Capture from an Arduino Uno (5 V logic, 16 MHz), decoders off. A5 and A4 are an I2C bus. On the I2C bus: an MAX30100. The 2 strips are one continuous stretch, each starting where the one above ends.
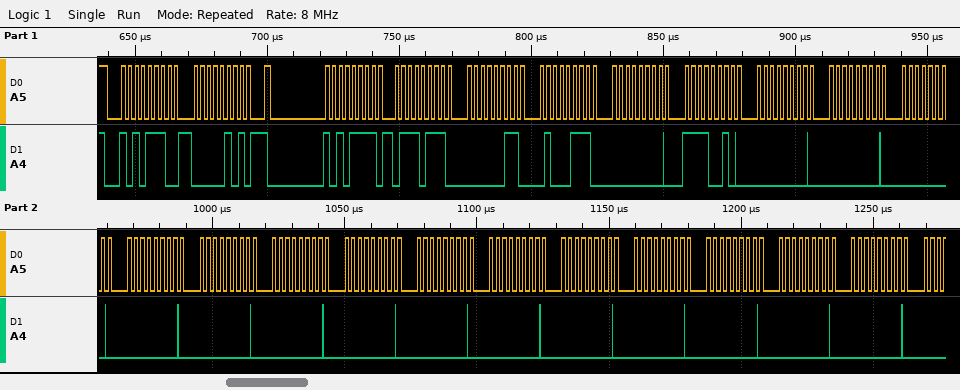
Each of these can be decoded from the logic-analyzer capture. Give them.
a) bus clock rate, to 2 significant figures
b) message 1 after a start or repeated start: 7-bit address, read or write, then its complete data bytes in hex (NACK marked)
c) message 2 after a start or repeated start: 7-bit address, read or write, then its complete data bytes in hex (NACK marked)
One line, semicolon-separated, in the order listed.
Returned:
400 kHz; 0x57 write: 05; 0x57 read: 77 03 47 00 F2 00 00 00 00 00 00 00 00 00 00 00 00 00 00
